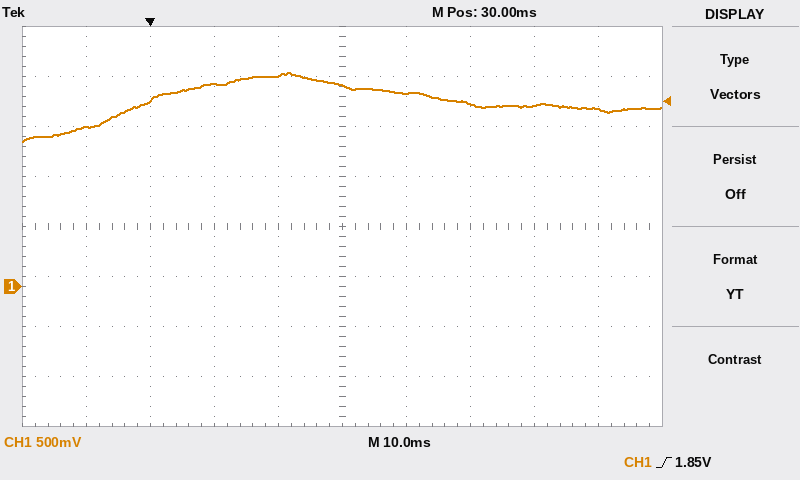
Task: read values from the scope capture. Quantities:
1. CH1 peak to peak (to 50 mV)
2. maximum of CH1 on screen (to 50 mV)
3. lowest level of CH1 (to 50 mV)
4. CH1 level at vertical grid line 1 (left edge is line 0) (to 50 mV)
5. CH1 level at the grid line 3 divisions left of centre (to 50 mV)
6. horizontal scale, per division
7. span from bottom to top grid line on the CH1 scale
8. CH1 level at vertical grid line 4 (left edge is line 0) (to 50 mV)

700 mV
2.15 V
1.45 V
1.60 V
1.85 V
10 ms
4 V
2.10 V
